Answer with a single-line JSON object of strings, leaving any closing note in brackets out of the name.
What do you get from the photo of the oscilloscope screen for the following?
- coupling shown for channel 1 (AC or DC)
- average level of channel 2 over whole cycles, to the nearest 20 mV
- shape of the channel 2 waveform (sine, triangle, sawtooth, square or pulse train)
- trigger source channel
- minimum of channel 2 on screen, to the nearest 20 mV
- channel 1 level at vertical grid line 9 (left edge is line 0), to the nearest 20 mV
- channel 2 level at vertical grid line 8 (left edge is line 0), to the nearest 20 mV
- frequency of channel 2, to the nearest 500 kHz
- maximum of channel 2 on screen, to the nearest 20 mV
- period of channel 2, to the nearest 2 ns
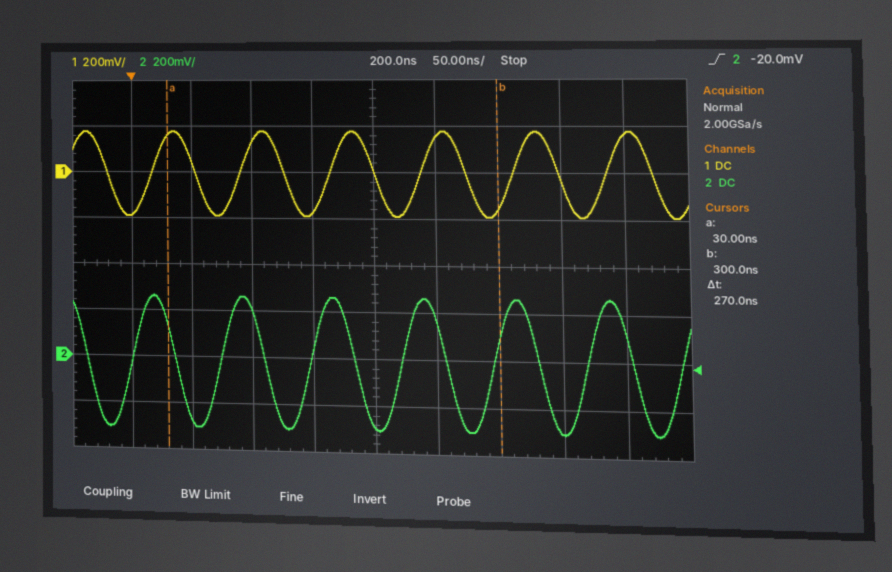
{"coupling shown for channel 1": "DC", "average level of channel 2 over whole cycles, to the nearest 20 mV": "-20 mV", "shape of the channel 2 waveform": "sine", "trigger source channel": "channel 2", "minimum of channel 2 on screen, to the nearest 20 mV": "-300 mV", "channel 1 level at vertical grid line 9 (left edge is line 0), to the nearest 20 mV": "160 mV", "channel 2 level at vertical grid line 8 (left edge is line 0), to the nearest 20 mV": "-300 mV", "frequency of channel 2, to the nearest 500 kHz": "13.5 MHz", "maximum of channel 2 on screen, to the nearest 20 mV": "260 mV", "period of channel 2, to the nearest 2 ns": "74 ns"}
